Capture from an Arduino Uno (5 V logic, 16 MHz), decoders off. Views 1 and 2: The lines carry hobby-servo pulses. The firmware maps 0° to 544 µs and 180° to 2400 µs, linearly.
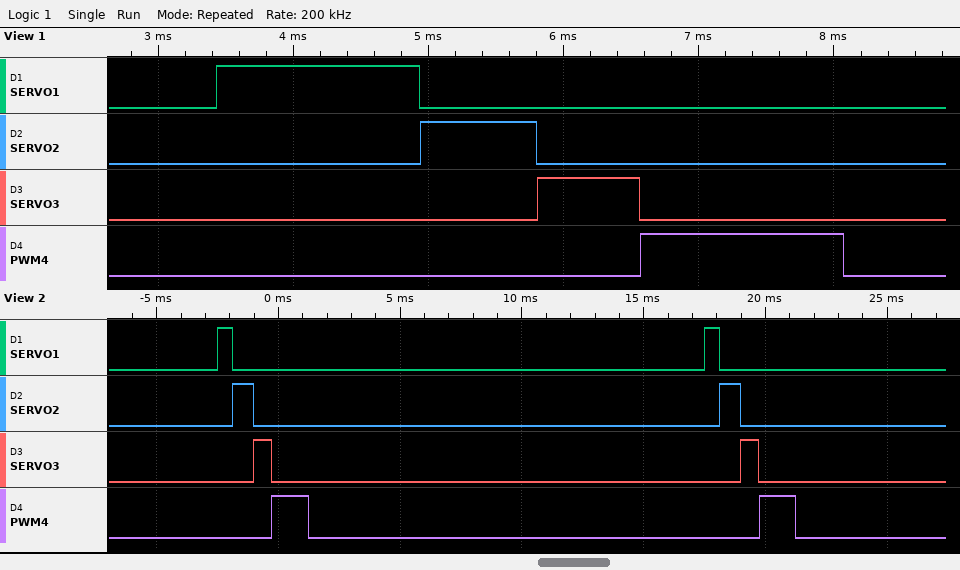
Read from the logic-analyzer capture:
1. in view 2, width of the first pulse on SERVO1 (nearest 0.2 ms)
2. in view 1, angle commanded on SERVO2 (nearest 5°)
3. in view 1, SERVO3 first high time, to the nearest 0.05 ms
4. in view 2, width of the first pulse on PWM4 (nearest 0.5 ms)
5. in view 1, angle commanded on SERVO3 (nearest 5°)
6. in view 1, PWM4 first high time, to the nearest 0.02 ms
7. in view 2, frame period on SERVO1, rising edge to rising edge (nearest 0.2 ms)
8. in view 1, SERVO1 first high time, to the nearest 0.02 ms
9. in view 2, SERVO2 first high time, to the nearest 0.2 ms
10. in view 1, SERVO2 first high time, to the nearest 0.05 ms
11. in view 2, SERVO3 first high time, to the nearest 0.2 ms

0.6 ms
30°
0.75 ms
1.5 ms
20°
1.50 ms
20.0 ms
1.50 ms
0.8 ms
0.85 ms
0.8 ms
